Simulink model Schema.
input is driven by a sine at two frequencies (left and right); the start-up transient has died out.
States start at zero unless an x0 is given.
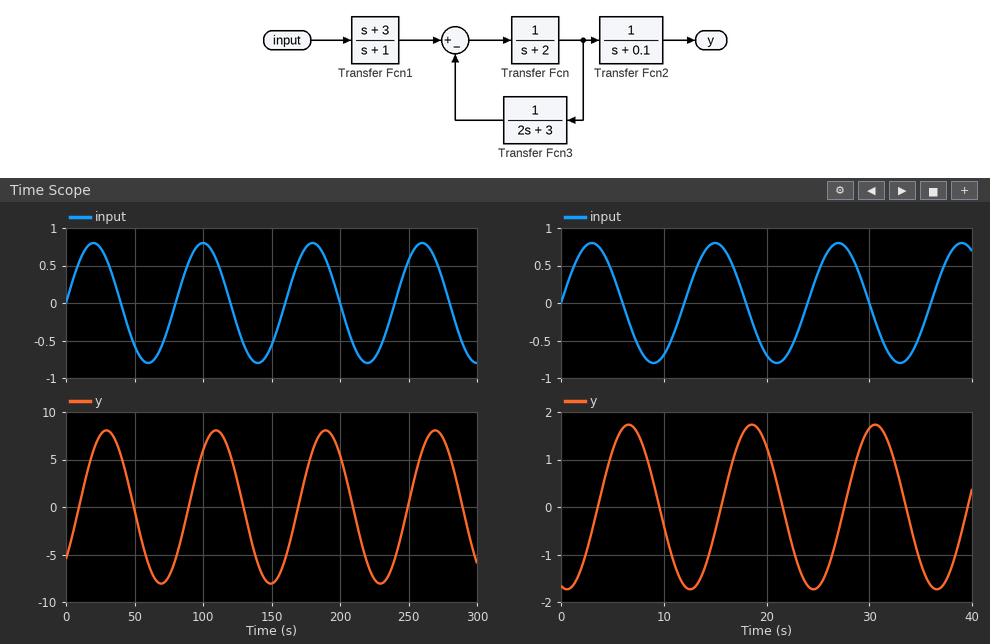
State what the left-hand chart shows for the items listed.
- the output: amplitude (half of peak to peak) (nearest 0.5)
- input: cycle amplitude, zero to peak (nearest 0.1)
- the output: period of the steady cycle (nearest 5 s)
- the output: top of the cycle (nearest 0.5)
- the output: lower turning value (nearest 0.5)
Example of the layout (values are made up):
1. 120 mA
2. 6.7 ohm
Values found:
1. 8.0
2. 0.8
3. 80 s
4. 8.0
5. -8.0
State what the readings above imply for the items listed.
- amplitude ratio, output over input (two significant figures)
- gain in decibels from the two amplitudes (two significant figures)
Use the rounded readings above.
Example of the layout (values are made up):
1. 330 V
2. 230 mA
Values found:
1. 10
2. 20 dB
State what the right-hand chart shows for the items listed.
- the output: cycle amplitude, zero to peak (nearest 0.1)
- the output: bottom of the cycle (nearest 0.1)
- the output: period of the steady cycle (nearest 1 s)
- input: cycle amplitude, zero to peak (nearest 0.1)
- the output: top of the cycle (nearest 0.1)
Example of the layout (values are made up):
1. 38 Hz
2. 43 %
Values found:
1. 1.7
2. -1.7
3. 12 s
4. 0.8
5. 1.7
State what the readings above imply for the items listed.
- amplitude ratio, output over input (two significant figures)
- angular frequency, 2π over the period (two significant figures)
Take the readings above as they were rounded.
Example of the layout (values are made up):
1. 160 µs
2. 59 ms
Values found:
1. 2.1
2. 0.52 rad/s
